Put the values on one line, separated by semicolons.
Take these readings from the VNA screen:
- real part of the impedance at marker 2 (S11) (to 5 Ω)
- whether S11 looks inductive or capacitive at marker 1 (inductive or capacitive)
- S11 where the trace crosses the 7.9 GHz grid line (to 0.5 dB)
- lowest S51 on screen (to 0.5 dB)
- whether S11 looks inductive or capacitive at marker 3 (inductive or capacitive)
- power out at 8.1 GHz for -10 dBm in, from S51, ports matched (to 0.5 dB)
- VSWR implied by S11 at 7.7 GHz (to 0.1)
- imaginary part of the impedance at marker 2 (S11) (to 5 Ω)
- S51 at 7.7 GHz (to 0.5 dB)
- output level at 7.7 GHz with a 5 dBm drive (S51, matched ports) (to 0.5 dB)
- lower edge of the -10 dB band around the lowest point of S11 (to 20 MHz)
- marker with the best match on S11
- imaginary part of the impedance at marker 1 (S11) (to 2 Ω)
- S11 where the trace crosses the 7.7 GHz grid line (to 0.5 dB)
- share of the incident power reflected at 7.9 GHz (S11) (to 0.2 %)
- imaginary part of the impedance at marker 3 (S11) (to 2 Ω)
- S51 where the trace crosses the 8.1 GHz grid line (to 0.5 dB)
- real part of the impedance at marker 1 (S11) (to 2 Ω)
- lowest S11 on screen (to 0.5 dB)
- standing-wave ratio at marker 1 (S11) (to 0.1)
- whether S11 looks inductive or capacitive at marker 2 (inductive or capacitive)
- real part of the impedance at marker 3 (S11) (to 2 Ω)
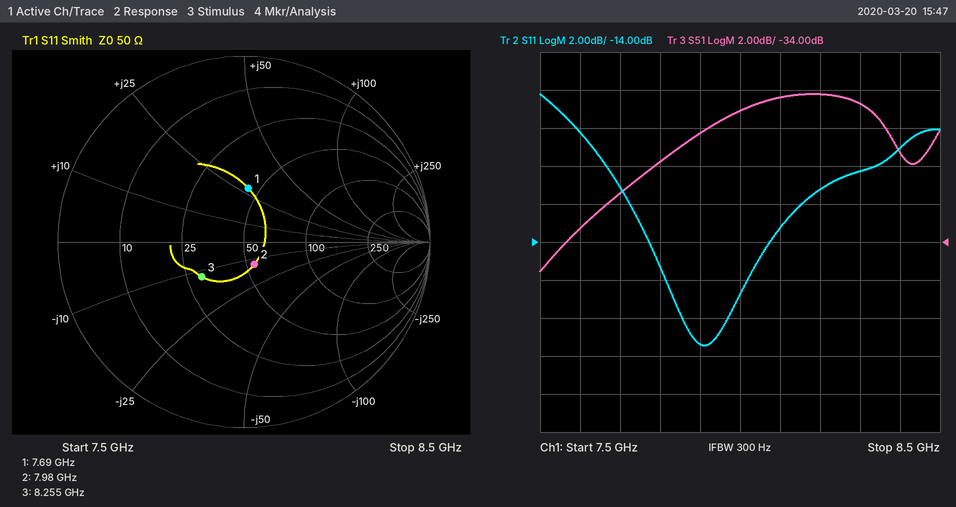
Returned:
55 Ω; inductive; -19.5 dB; -35.5 dB; capacitive; -36.5 dBm; 1.8; -15 Ω; -31.5 dB; -26.5 dBm; 7.66 GHz; marker 2; +28 Ω; -11.0 dB; 1.2 %; -12 Ω; -26.5 dB; 44 Ω; -19.5 dB; 1.8; capacitive; 30 Ω
